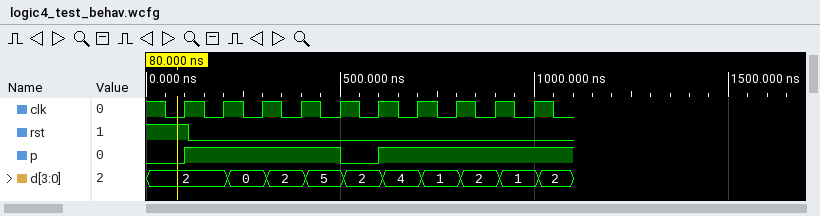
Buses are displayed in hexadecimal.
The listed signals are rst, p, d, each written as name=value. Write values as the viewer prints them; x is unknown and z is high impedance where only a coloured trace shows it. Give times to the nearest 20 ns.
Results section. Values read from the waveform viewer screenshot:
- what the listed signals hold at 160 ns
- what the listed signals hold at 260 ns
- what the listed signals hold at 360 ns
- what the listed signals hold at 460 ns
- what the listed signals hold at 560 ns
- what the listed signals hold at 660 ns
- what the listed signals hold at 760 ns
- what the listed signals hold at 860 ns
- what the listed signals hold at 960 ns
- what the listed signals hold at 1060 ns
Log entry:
rst=0, p=1, d=2
rst=0, p=1, d=0
rst=0, p=1, d=2
rst=0, p=1, d=5
rst=0, p=0, d=2
rst=0, p=1, d=4
rst=0, p=1, d=1
rst=0, p=1, d=2
rst=0, p=1, d=1
rst=0, p=1, d=2
